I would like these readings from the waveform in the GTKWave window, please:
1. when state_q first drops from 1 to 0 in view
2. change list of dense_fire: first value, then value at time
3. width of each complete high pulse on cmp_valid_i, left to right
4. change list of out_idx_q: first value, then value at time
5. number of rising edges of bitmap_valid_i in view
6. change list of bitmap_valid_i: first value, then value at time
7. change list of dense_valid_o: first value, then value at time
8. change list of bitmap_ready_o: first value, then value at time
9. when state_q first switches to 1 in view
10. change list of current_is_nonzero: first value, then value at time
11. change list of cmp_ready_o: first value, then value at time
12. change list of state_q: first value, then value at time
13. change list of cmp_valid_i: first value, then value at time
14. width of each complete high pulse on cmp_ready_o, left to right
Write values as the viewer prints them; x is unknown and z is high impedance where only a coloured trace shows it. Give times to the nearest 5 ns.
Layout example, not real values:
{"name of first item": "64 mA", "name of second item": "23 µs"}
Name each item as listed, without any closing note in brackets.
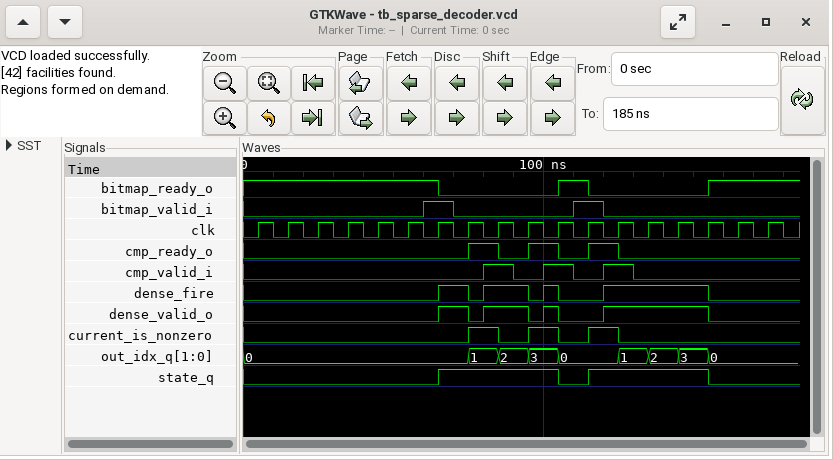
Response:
{"when state_q first drops from 1 to 0 in view": "105 ns", "change list of dense_fire: first value, then value at time": "0, 1 at 65 ns, 0 at 75 ns, 1 at 80 ns, 0 at 95 ns, 1 at 100 ns, 0 at 105 ns, 1 at 120 ns, 0 at 155 ns", "width of each complete high pulse on cmp_valid_i, left to right": "10 ns, 10 ns, 10 ns", "change list of out_idx_q: first value, then value at time": "0, 1 at 75 ns, 2 at 85 ns, 3 at 95 ns, 0 at 105 ns, 1 at 125 ns, 2 at 135 ns, 3 at 145 ns, 0 at 155 ns", "number of rising edges of bitmap_valid_i in view": "2", "change list of bitmap_valid_i: first value, then value at time": "0, 1 at 60 ns, 0 at 70 ns, 1 at 110 ns, 0 at 120 ns", "change list of dense_valid_o: first value, then value at time": "0, 1 at 65 ns, 0 at 75 ns, 1 at 80 ns, 0 at 95 ns, 1 at 100 ns, 0 at 105 ns, 1 at 120 ns, 0 at 155 ns", "change list of bitmap_ready_o: first value, then value at time": "1, 0 at 65 ns, 1 at 105 ns, 0 at 115 ns, 1 at 155 ns", "when state_q first switches to 1 in view": "65 ns", "change list of current_is_nonzero: first value, then value at time": "0, 1 at 75 ns, 0 at 85 ns, 1 at 95 ns, 0 at 105 ns, 1 at 115 ns, 0 at 125 ns", "change list of cmp_ready_o: first value, then value at time": "0, 1 at 75 ns, 0 at 85 ns, 1 at 95 ns, 0 at 105 ns, 1 at 115 ns, 0 at 125 ns", "change list of state_q: first value, then value at time": "0, 1 at 65 ns, 0 at 105 ns, 1 at 115 ns, 0 at 155 ns", "change list of cmp_valid_i: first value, then value at time": "0, 1 at 80 ns, 0 at 90 ns, 1 at 100 ns, 0 at 110 ns, 1 at 120 ns, 0 at 130 ns", "width of each complete high pulse on cmp_ready_o, left to right": "10 ns, 10 ns, 10 ns"}
